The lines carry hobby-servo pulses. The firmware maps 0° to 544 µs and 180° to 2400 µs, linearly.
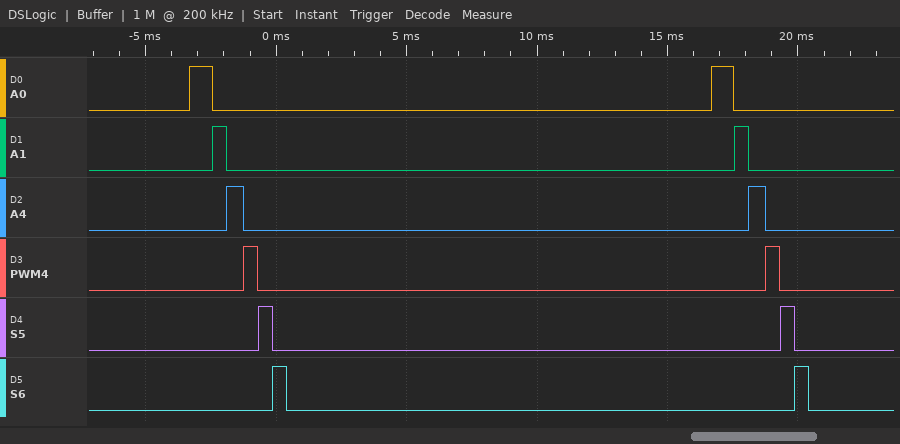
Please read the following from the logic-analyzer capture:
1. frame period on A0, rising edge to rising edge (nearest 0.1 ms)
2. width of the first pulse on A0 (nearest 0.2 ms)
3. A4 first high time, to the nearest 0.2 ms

20.0 ms
0.8 ms
0.6 ms
